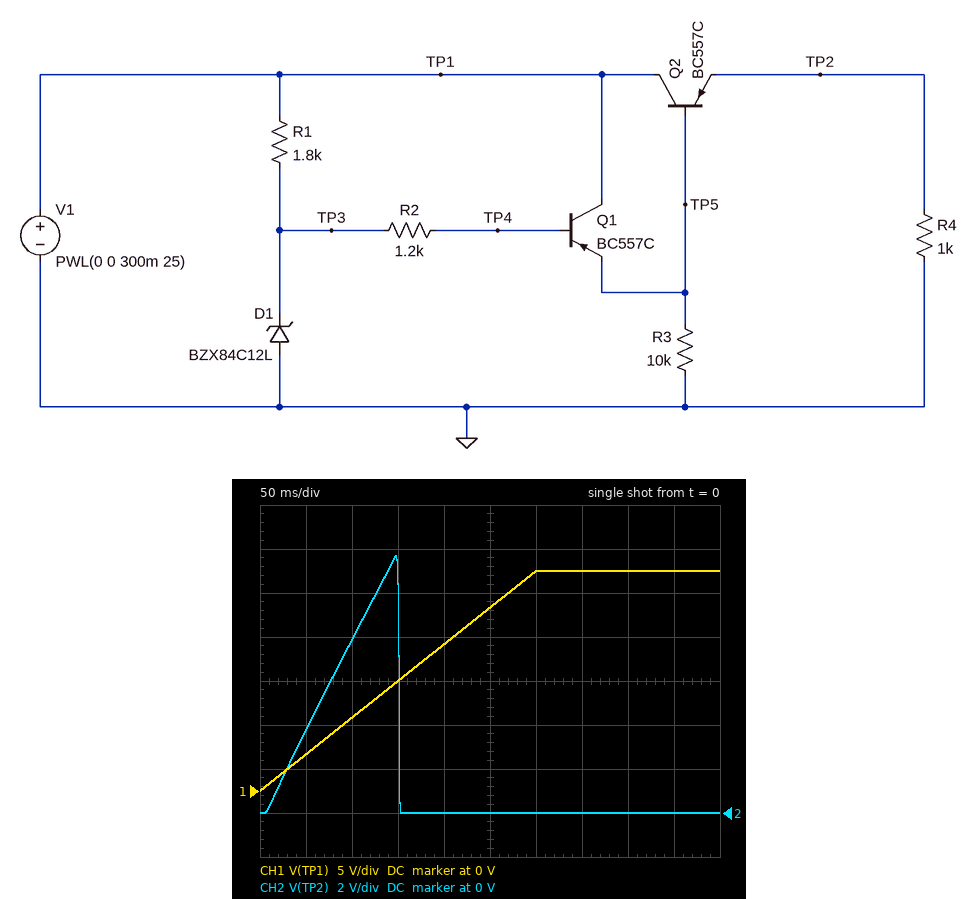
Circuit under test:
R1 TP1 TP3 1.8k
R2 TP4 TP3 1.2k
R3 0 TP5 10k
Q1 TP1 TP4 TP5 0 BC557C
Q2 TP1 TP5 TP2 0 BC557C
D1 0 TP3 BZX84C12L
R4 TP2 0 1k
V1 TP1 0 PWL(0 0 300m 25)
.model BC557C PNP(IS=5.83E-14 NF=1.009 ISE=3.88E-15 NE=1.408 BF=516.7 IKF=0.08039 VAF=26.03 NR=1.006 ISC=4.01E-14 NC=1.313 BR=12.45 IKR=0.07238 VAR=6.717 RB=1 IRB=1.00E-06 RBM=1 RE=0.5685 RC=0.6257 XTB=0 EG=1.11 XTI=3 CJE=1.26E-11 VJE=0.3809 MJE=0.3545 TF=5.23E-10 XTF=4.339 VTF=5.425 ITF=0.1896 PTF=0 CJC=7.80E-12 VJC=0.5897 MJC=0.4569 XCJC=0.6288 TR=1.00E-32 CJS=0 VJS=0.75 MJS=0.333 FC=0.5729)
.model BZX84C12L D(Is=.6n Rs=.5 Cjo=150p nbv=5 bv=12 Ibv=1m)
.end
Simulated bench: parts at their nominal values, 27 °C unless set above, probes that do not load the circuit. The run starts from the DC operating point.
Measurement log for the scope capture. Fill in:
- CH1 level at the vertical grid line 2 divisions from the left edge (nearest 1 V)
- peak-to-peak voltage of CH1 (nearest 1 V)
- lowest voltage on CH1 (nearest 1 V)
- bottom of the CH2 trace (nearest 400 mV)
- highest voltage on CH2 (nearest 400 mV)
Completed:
8 V
25 V
0 V
0 V
11.6 V
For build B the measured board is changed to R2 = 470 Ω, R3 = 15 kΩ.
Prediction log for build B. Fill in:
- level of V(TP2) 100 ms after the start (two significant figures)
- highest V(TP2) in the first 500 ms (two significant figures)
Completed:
6.6 V
10 V
